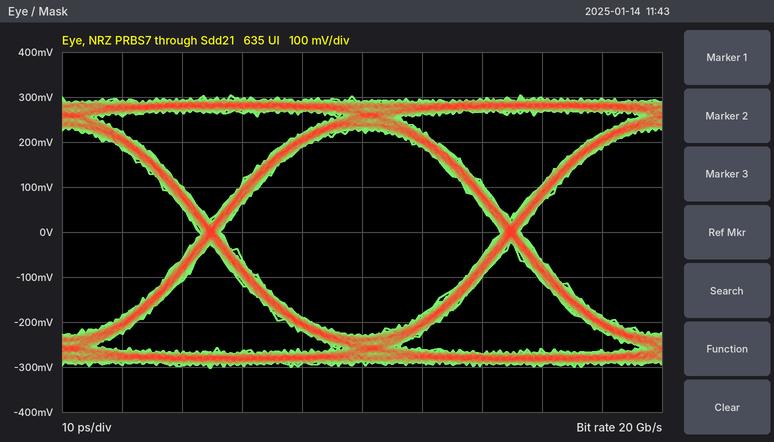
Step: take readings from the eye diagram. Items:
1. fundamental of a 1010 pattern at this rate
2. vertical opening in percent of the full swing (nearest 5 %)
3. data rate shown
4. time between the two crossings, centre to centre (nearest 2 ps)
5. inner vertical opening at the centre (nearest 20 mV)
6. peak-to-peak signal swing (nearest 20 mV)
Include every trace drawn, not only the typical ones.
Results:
10 GHz
75 %
20 Gb/s
50 ps
460 mV
600 mV
